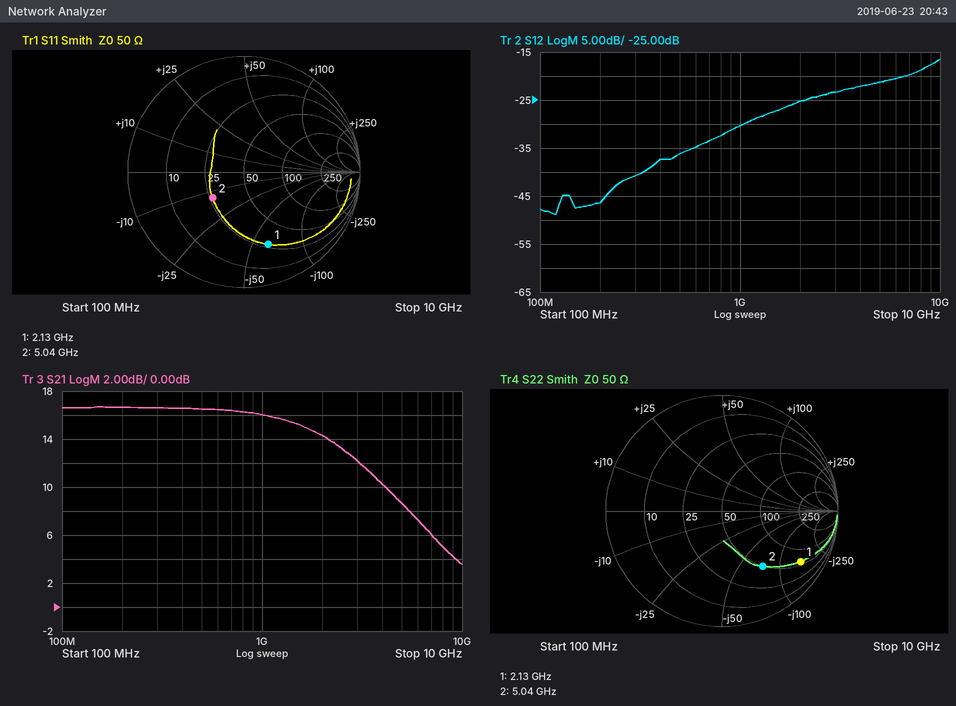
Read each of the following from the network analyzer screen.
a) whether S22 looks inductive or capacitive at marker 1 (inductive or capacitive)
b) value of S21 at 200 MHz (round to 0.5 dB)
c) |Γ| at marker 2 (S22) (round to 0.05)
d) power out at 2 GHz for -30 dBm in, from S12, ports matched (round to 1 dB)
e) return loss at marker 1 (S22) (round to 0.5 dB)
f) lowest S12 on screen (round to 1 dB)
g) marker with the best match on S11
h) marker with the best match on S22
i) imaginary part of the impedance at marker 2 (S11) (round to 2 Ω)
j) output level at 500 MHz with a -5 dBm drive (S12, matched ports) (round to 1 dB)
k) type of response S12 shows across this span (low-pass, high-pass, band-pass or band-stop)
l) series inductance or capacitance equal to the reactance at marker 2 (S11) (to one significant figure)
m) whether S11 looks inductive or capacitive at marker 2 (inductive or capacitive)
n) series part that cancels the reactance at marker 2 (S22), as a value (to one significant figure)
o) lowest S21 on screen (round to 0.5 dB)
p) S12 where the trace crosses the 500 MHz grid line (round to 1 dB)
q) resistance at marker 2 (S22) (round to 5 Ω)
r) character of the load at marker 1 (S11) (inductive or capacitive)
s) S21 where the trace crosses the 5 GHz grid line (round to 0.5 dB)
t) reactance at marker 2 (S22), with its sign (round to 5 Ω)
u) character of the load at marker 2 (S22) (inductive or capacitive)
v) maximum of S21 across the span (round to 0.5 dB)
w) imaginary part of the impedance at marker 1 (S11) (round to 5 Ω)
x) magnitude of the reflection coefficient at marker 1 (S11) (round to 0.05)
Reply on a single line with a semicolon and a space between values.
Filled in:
capacitive; 16.5 dB; 0.60; -55 dBm; 2.0 dB; -49 dB; marker 2; marker 2; -14 Ω; -41 dBm; high-pass; 2 pF; capacitive; 2 nH; 3.5 dB; -36 dB; 50 Ω; capacitive; 8.5 dB; -75 Ω; capacitive; 16.5 dB; -60 Ω; 0.65
